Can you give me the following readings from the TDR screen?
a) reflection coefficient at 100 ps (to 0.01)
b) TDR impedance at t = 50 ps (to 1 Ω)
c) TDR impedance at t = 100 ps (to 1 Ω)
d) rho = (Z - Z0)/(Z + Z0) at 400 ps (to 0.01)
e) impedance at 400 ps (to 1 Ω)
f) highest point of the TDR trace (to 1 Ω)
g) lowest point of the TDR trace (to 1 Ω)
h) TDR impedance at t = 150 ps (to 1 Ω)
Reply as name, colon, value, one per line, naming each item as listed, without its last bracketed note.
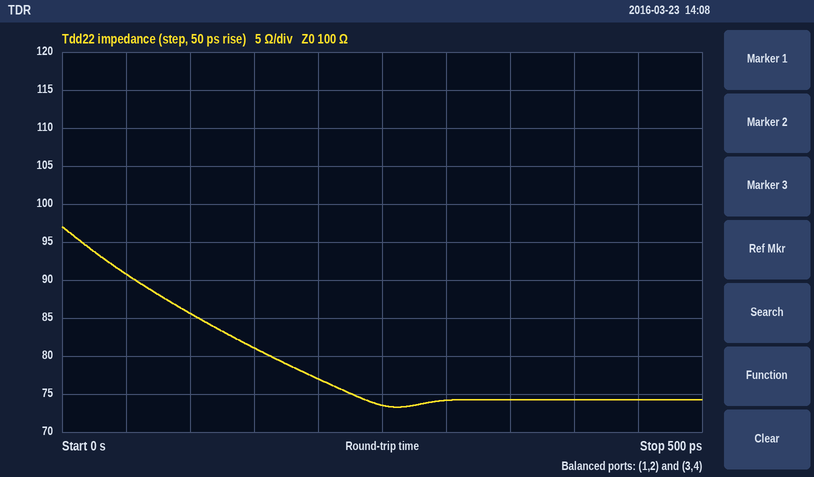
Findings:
reflection coefficient at 100 ps: -0.08
TDR impedance at t = 50 ps: 91 Ω
TDR impedance at t = 100 ps: 86 Ω
rho = (Z - Z0)/(Z + Z0) at 400 ps: -0.15
impedance at 400 ps: 74 Ω
highest point of the TDR trace: 97 Ω
lowest point of the TDR trace: 73 Ω
TDR impedance at t = 150 ps: 81 Ω
